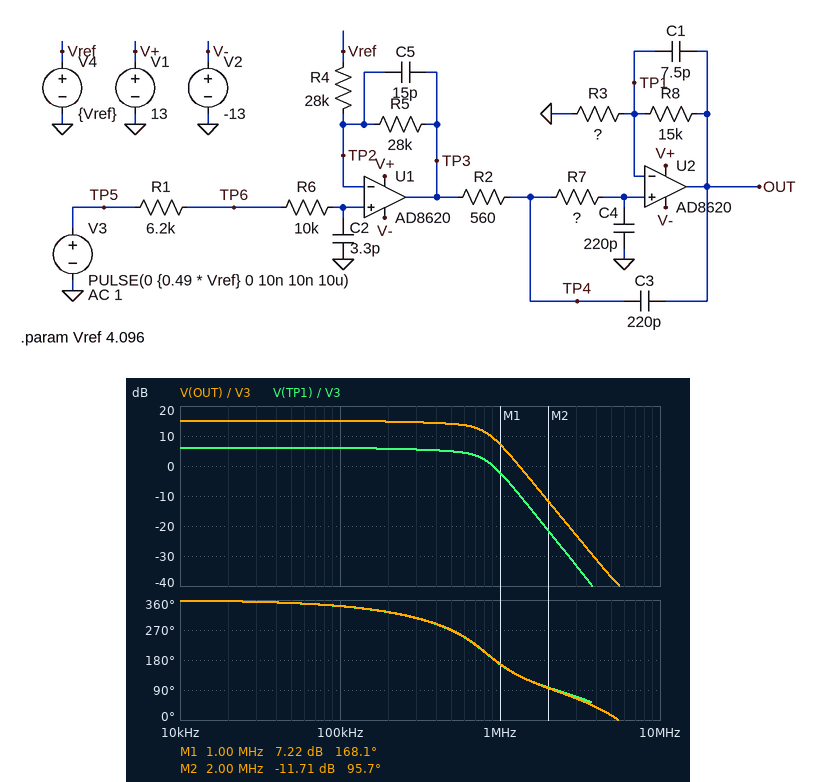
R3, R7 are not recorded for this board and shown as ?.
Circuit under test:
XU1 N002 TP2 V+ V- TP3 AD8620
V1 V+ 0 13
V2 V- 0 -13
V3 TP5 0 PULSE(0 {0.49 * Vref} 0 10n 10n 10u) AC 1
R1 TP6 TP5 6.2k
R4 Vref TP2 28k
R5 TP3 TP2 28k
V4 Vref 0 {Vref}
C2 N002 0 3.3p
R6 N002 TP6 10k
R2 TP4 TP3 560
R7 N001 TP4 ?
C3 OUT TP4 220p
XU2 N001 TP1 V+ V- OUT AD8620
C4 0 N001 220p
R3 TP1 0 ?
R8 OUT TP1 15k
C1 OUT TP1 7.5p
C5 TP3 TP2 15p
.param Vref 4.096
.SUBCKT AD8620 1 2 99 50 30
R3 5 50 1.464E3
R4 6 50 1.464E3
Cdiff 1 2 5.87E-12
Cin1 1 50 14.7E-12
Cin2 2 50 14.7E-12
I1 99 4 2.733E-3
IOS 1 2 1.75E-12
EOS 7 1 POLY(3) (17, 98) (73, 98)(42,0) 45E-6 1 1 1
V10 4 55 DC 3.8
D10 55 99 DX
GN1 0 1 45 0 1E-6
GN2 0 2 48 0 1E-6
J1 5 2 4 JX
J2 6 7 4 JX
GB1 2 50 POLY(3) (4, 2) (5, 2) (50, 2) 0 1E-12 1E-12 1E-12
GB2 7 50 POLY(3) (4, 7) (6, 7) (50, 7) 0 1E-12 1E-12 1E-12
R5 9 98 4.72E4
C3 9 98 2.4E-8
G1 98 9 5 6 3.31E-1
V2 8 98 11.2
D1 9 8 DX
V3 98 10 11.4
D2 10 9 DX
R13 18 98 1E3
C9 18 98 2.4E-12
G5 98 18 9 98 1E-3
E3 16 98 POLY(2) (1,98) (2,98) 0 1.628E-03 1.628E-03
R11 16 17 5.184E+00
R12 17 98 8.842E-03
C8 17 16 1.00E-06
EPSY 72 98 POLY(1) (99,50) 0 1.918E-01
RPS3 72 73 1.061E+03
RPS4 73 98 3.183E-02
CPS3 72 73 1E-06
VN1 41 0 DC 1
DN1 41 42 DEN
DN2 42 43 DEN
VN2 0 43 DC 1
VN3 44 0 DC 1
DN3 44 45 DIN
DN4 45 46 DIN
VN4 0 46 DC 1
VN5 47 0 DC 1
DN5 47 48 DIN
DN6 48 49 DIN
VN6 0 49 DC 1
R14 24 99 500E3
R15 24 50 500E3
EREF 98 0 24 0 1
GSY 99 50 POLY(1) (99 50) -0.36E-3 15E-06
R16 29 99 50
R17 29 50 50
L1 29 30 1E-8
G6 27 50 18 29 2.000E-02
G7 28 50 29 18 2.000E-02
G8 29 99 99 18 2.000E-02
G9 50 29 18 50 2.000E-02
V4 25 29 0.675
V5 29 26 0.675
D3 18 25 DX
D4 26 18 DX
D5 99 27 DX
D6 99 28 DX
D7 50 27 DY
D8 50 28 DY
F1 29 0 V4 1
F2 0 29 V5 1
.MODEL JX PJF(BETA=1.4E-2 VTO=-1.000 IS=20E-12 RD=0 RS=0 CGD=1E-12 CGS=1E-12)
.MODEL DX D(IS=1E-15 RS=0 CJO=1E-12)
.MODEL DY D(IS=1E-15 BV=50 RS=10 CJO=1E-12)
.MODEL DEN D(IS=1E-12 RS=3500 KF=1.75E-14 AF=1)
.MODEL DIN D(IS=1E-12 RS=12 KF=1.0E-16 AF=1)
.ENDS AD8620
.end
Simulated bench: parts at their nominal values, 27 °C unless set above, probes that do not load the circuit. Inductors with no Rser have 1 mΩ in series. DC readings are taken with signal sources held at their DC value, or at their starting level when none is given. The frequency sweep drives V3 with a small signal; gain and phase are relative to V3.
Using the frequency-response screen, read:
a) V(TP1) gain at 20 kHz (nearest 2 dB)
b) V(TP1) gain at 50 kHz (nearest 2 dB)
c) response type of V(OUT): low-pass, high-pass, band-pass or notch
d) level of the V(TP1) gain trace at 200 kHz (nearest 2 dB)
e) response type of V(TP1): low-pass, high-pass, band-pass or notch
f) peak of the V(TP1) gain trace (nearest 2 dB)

6 dB
6 dB
low-pass
6 dB
low-pass
6 dB
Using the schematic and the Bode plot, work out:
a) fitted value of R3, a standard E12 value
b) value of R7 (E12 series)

8.2 kΩ
1.2 kΩ
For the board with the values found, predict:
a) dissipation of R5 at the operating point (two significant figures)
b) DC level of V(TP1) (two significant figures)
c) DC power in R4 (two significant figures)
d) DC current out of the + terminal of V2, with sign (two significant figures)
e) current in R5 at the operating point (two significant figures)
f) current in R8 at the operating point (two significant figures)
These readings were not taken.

600 µW
-4.1 V
600 µW
-6.2 mA
150 µA
500 µA
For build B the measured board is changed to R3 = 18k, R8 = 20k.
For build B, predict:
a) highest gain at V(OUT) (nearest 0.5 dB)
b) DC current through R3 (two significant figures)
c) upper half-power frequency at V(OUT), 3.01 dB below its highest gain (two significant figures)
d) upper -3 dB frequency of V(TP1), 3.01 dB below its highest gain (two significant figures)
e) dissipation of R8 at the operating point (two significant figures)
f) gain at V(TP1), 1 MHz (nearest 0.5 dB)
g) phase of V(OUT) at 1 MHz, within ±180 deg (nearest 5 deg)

12.5 dB
230 µA
580 kHz
470 kHz
1.0 mW
-2.5 dB
-165 deg
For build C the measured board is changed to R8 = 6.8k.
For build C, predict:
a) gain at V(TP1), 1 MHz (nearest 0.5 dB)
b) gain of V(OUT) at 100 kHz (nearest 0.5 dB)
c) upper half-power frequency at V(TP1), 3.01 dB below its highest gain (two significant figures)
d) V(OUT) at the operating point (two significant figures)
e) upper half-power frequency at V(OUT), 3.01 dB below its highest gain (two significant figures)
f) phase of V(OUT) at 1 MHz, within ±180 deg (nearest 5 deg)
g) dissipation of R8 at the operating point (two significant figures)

-5.5 dB
11.0 dB
420 kHz
-7.5 V
430 kHz
-160 deg
1.7 mW
